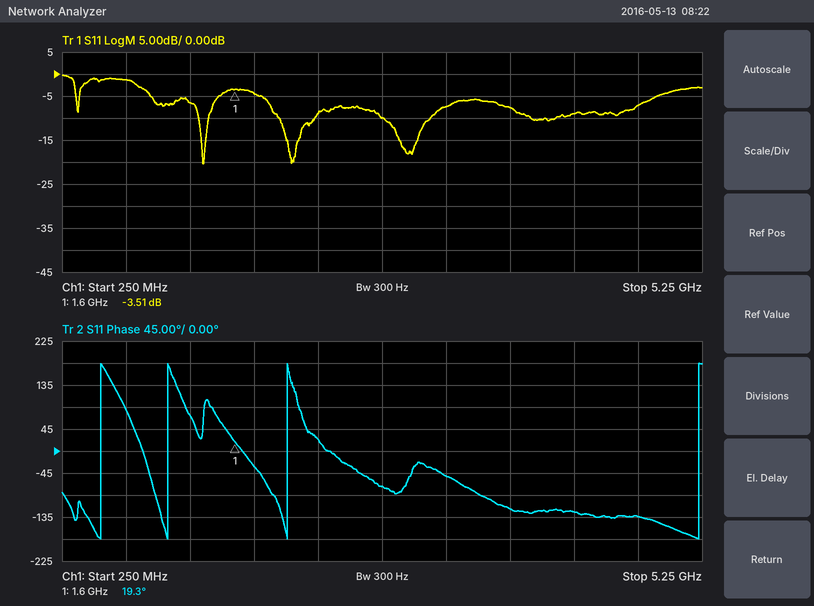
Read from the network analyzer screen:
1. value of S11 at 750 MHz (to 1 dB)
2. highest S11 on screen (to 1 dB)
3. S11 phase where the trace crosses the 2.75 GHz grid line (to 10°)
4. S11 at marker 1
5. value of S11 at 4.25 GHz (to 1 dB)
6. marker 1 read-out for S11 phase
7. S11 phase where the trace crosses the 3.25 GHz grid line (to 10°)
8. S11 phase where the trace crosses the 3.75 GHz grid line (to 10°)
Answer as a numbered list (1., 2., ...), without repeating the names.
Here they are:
1. -1 dB
2. 0 dB
3. -70°
4. -3.51 dB
5. -9 dB
6. 19.3°
7. -50°
8. -120°
